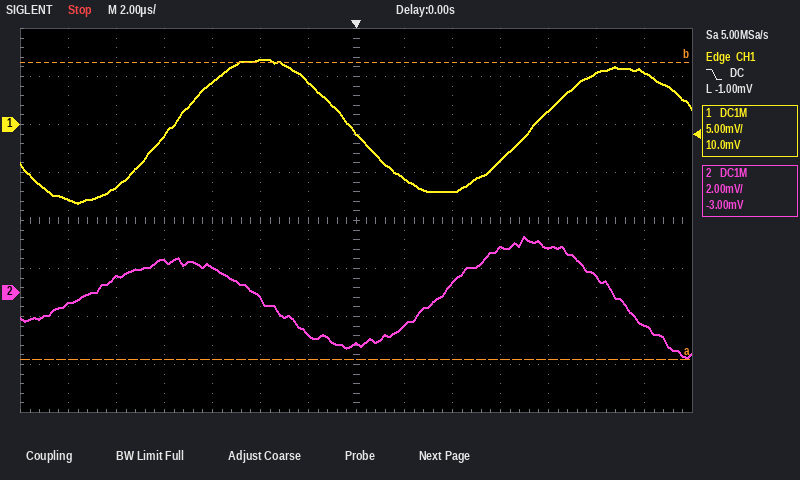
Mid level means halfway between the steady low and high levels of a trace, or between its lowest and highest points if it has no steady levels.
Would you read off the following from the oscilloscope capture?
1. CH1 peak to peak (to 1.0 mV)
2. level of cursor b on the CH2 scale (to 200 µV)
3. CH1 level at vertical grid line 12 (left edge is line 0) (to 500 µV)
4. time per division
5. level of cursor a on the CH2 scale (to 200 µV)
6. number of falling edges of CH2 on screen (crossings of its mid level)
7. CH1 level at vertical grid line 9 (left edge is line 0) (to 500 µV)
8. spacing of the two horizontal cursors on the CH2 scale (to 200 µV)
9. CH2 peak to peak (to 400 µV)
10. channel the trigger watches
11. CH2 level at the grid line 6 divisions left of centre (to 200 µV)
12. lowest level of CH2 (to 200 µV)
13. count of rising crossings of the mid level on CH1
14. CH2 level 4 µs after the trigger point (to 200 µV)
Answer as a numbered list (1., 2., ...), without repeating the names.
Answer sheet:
1. 15.0 mV
2. 9.6 mV
3. 5.5 mV
4. 2 µs
5. -2.8 mV
6. 2
7. -7.0 mV
8. 12.4 mV
9. 5.2 mV
10. CH1
11. -400 µV
12. -2.8 mV
13. 2
14. 400 µV
